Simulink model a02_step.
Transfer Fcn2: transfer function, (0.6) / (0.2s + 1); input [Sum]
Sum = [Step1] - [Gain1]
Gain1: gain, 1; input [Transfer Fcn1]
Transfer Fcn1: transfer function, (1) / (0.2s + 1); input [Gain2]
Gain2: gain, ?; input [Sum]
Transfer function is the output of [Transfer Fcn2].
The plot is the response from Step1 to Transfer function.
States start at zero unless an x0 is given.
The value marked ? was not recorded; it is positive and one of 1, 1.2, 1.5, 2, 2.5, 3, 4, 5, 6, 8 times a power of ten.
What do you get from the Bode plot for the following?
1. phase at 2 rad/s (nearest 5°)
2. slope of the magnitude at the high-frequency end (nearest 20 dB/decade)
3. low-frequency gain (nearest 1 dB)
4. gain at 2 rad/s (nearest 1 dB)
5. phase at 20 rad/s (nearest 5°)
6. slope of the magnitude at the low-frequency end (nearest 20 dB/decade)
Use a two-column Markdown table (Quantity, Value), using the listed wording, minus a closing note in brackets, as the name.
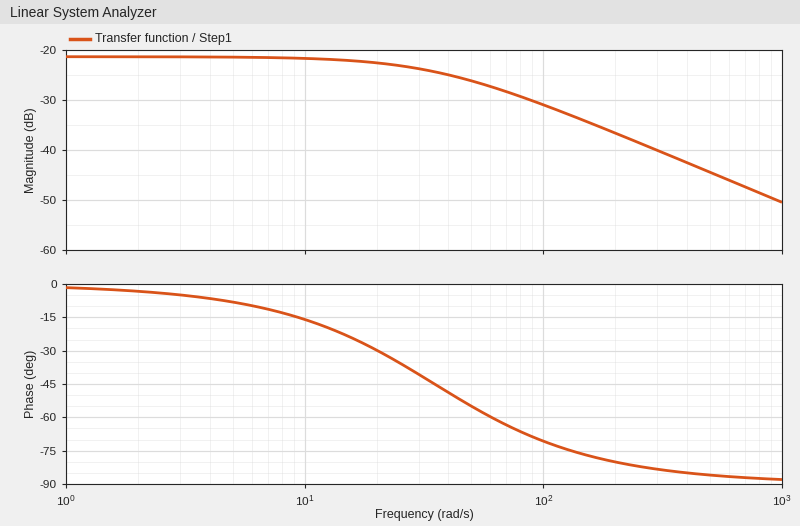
| Quantity | Value |
|---|---|
| phase at 2 rad/s | -5° |
| slope of the magnitude at the high-frequency end | -20 dB/decade |
| low-frequency gain | -21 dB |
| gain at 2 rad/s | -21 dB |
| phase at 20 rad/s | -30° |
| slope of the magnitude at the low-frequency end | 0 dB/decade |
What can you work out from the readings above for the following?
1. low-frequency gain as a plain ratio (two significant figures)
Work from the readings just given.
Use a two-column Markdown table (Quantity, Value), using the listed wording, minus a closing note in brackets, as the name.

| Quantity | Value |
|---|---|
| low-frequency gain as a plain ratio | 0.089 |
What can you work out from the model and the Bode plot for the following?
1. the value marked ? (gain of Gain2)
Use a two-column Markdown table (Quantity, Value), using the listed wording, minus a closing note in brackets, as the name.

| Quantity | Value |
|---|---|
| the value marked ? | 6 |
